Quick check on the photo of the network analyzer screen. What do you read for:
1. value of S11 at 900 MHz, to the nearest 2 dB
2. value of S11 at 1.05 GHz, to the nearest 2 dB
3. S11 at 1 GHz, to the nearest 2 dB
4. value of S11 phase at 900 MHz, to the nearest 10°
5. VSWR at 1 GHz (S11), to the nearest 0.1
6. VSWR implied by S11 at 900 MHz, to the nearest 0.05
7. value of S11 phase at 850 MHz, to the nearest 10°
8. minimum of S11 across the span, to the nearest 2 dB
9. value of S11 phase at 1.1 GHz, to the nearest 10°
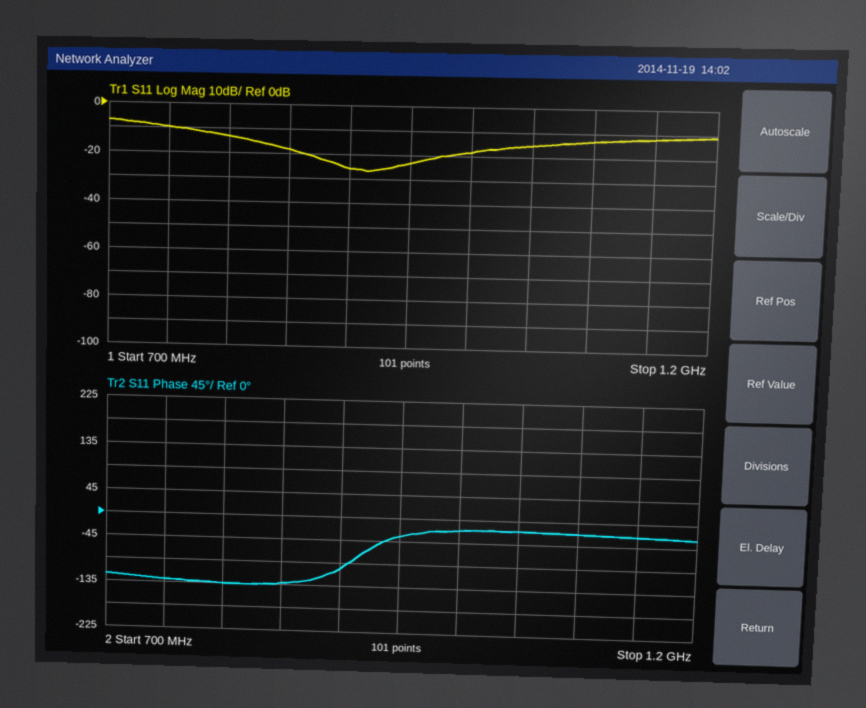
-26 dB
-16 dB
-18 dB
-100°
1.3
1.10
-130°
-26 dB
-20°
